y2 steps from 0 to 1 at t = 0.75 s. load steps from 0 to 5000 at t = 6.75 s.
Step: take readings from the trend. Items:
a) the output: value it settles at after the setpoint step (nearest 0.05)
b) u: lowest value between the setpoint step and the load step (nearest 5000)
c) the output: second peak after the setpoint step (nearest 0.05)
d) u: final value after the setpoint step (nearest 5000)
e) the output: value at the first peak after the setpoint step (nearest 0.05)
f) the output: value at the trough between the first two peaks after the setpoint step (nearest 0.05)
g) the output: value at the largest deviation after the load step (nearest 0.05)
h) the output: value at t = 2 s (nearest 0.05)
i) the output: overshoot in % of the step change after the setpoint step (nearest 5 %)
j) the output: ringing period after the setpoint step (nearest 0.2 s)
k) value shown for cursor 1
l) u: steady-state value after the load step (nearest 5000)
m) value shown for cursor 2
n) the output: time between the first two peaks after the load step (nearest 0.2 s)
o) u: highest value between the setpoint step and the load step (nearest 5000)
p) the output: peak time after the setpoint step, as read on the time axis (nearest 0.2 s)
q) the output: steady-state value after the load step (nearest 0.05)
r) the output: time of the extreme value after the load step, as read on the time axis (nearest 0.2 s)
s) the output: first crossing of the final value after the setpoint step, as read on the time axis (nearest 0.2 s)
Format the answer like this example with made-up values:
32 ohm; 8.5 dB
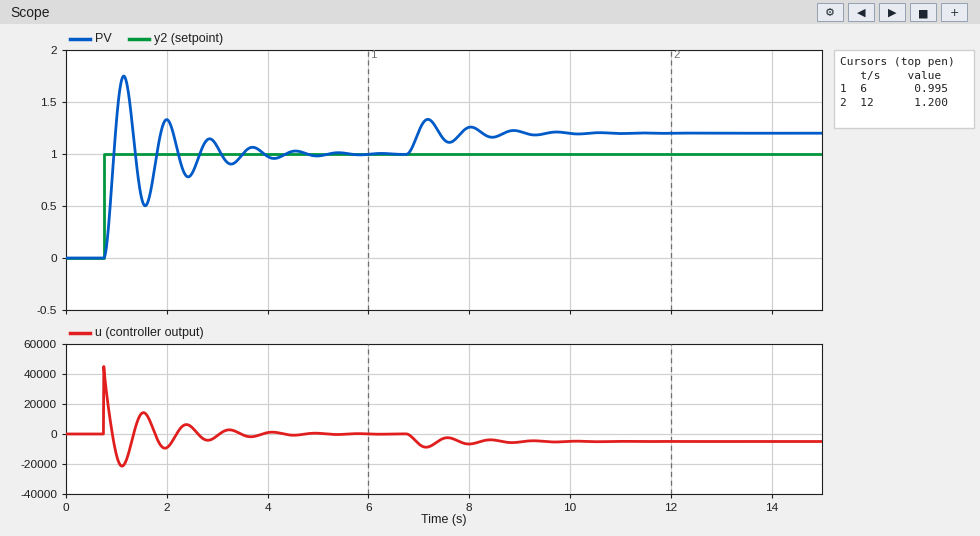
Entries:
1.00; -20000; 1.35; 0; 1.75; 0.50; 1.35; 1.35; 75 %; 0.8 s; 0.995; -5000; 1.200; 0.8 s; 45000; 1.2 s; 1.20; 7.2 s; 1.0 s
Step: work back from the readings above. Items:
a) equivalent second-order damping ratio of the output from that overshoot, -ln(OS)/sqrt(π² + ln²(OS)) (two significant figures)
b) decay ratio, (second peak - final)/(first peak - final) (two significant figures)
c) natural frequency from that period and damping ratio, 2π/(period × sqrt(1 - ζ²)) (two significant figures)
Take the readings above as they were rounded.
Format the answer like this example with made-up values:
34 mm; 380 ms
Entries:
0.091; 0.47; 7.9 rad/s
